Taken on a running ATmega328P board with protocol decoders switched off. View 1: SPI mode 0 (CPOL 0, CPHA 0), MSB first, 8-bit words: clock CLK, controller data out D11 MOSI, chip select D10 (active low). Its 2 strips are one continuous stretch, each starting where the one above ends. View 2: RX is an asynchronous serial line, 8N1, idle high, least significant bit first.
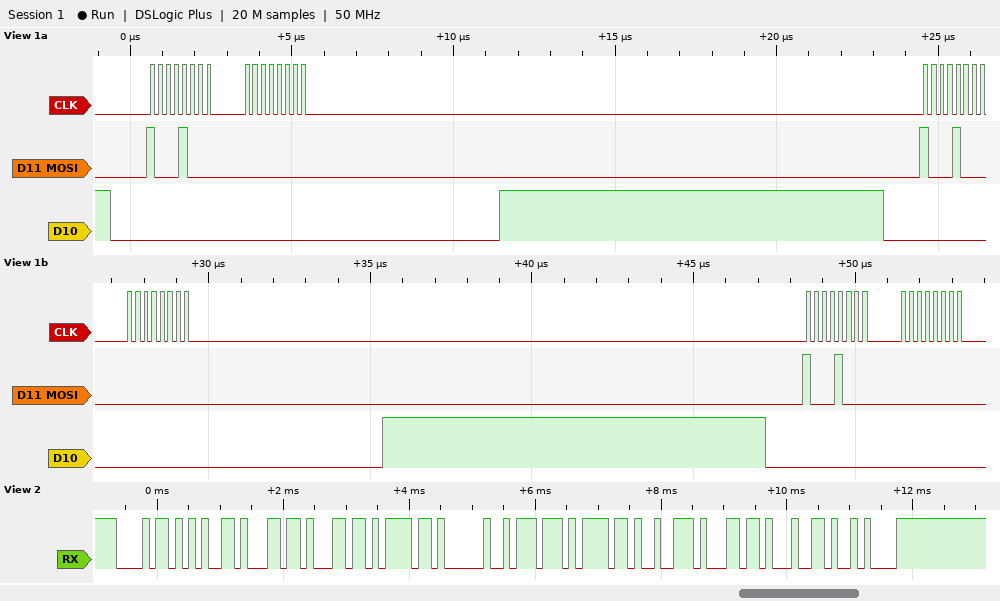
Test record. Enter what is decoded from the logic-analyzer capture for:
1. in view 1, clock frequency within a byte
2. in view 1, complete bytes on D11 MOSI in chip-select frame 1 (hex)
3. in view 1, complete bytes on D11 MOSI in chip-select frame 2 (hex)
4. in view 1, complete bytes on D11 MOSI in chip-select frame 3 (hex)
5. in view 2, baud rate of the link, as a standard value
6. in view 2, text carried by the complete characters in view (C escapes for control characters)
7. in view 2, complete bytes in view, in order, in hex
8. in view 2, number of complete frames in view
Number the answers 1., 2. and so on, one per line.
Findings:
1. 4 MHz
2. 88 00
3. 88 00
4. 88 00
5. 9600 baud
6. "hello world\n"
7. 0x68 0x65 0x6C 0x6C 0x6F 0x20 0x77 0x6F 0x72 0x6C 0x64 0x0A
8. 12
